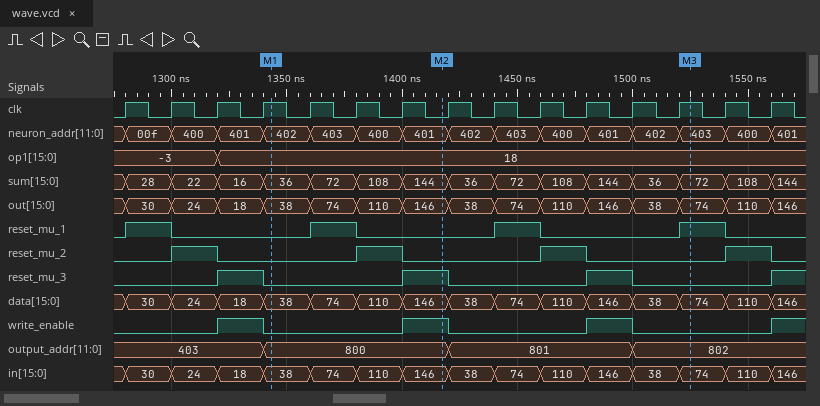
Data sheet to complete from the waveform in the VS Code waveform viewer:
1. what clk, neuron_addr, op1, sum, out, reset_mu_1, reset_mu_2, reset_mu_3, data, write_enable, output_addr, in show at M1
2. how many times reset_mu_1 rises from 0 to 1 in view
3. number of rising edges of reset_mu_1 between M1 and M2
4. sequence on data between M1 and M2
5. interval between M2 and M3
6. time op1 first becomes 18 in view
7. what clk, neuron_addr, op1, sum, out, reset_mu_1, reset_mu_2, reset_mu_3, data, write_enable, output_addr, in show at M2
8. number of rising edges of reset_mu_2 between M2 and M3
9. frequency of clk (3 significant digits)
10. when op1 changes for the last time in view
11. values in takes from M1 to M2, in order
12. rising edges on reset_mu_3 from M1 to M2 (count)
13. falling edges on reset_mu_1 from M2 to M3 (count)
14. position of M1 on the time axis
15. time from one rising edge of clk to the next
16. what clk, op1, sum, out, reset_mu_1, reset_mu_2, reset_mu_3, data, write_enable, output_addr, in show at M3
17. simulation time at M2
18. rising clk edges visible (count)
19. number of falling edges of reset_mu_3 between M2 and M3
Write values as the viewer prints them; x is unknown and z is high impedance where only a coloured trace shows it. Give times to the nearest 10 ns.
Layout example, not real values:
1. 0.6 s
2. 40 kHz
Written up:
1. clk=1, neuron_addr=402, op1=18, sum=36, out=38, reset_mu_1=0, reset_mu_2=0, reset_mu_3=0, data=38, write_enable=0, output_addr=800, in=38
2. 4
3. 1
4. 38, 74, 110, 146
5. 110 ns
6. 1320 ns
7. clk=0, neuron_addr=401, op1=18, sum=144, out=146, reset_mu_1=0, reset_mu_2=0, reset_mu_3=1, data=146, write_enable=1, output_addr=800, in=146
8. 1
9. 50.0 MHz
10. 1320 ns
11. 38, 74, 110, 146
12. 1
13. 1
14. 1340 ns
15. 20 ns
16. clk=1, op1=18, sum=72, out=74, reset_mu_1=1, reset_mu_2=0, reset_mu_3=0, data=74, write_enable=0, output_addr=802, in=74
17. 1420 ns
18. 15
19. 2
